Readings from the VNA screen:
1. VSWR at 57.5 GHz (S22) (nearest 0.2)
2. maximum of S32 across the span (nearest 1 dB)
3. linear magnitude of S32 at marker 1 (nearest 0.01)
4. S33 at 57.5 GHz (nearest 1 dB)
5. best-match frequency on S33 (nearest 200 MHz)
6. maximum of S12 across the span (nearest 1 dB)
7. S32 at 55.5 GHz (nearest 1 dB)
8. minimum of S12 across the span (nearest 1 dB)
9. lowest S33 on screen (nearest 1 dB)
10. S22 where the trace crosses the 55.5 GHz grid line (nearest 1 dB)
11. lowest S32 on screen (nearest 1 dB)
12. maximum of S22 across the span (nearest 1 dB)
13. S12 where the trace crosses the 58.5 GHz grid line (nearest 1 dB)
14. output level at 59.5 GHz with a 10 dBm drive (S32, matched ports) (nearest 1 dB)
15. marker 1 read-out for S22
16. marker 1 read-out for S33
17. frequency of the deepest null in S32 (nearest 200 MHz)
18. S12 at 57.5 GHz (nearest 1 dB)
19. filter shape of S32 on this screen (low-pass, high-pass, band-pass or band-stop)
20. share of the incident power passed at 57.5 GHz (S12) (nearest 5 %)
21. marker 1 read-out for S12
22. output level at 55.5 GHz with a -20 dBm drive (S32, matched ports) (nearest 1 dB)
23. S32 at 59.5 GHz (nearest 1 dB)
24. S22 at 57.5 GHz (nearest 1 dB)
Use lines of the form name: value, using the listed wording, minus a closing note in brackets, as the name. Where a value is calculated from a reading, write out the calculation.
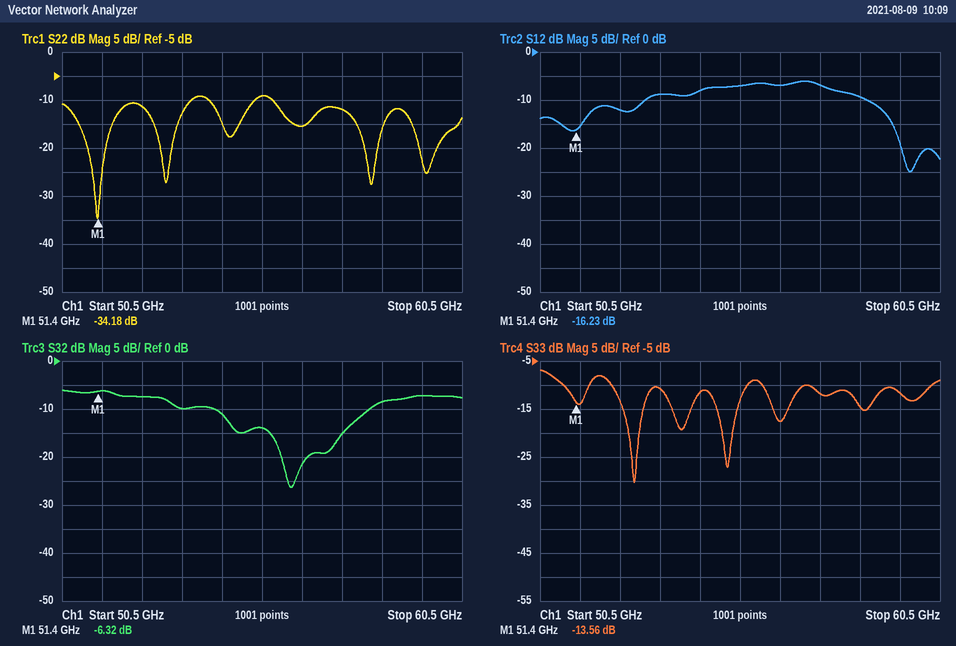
VSWR at 57.5 GHz (S22): |Γ| = 10^(-12/20) = 0.2512; VSWR = (1 + 0.2512)/(1 − 0.2512) ≈ 1.67, so 1.6 to the nearest 0.2
maximum of S32 across the span: -6 dB
linear magnitude of S32 at marker 1: 10^(-6.32/20) ≈ 0.48
S33 at 57.5 GHz: -12 dB
best-match frequency on S33: 52.8 GHz
maximum of S12 across the span: -6 dB
S32 at 55.5 GHz: -14 dB
minimum of S12 across the span: -25 dB
lowest S33 on screen: -30 dB
S22 where the trace crosses the 55.5 GHz grid line: -9 dB
lowest S32 on screen: -26 dB
maximum of S22 across the span: -9 dB
S12 where the trace crosses the 58.5 GHz grid line: -9 dB
output level at 59.5 GHz with a 10 dBm drive (S32, matched ports): 10 dBm + (-7 dB) = 3 dBm
marker 1 read-out for S22: -34.18 dB
marker 1 read-out for S33: -13.56 dB
frequency of the deepest null in S32: 56.2 GHz
S12 at 57.5 GHz: -7 dB
filter shape of S32 on this screen: band-stop
share of the incident power passed at 57.5 GHz (S12): 10^(-7/10) ≈ 20 %
marker 1 read-out for S12: -16.23 dB
output level at 55.5 GHz with a -20 dBm drive (S32, matched ports): -20 dBm + (-14 dB) = -34 dBm
S32 at 59.5 GHz: -7 dB
S22 at 57.5 GHz: -12 dB
